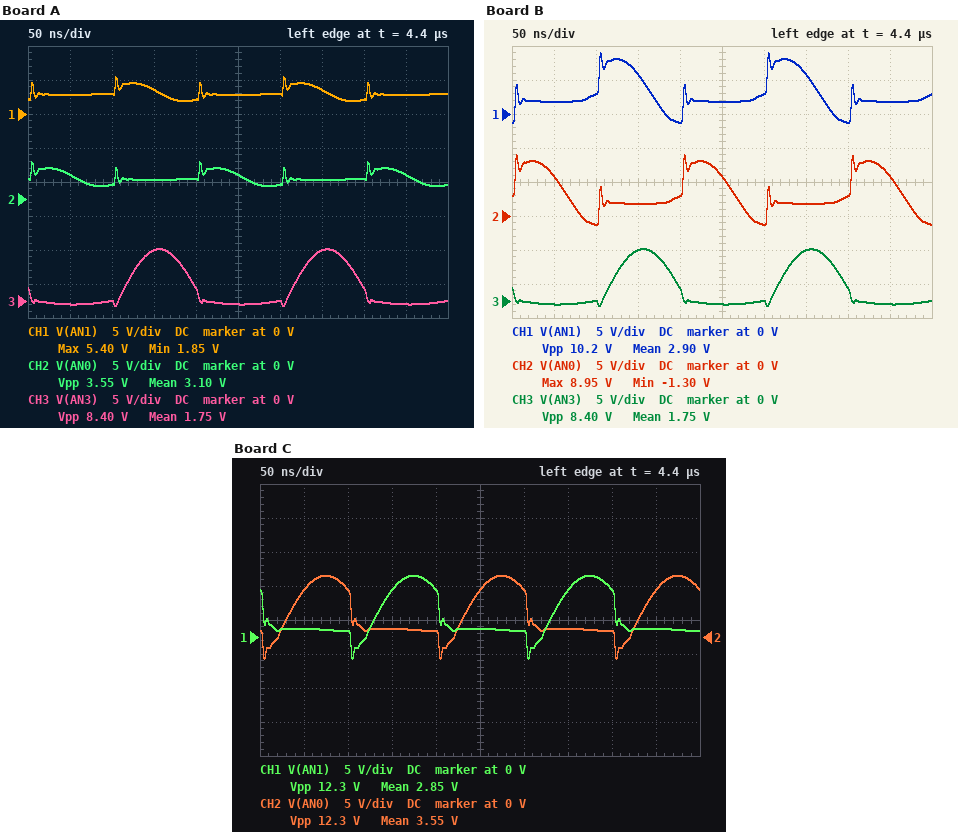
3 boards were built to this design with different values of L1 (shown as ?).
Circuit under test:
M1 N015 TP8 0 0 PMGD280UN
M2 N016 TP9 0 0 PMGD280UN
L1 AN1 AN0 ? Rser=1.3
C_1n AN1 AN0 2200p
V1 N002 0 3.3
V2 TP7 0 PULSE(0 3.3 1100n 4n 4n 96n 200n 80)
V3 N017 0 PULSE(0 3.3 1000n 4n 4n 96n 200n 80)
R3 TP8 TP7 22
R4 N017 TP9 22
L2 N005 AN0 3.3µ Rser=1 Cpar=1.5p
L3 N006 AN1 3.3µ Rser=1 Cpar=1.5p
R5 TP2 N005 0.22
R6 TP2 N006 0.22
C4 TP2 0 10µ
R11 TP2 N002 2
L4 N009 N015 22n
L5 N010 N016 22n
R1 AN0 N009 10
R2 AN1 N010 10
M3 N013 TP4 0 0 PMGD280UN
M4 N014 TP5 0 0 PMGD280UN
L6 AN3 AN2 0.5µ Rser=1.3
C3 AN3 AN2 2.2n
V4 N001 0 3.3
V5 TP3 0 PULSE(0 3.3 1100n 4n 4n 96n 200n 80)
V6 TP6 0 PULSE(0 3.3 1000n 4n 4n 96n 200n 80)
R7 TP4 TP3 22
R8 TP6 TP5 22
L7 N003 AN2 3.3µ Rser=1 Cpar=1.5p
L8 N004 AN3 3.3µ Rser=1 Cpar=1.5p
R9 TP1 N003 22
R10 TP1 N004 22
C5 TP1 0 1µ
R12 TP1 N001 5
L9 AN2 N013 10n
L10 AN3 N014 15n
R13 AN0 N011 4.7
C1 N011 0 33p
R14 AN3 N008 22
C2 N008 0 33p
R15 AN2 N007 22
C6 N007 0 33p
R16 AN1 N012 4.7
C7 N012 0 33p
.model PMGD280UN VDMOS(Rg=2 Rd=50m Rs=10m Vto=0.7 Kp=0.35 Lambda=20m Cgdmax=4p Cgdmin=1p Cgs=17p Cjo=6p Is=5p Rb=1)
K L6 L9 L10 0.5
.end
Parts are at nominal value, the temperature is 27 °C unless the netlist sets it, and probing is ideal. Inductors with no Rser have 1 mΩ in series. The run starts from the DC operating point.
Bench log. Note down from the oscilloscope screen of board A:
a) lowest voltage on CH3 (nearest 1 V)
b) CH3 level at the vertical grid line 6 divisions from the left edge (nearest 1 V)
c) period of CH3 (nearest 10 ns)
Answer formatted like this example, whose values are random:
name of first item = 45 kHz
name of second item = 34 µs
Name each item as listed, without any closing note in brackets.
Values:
lowest voltage on CH3 = -1 V
CH3 level at the vertical grid line 6 divisions from the left edge = 0 V
period of CH3 = 200 ns
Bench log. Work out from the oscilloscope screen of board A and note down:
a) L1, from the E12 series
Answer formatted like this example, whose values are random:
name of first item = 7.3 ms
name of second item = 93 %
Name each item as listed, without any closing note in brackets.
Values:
L1, from the E12 series = 180 nH
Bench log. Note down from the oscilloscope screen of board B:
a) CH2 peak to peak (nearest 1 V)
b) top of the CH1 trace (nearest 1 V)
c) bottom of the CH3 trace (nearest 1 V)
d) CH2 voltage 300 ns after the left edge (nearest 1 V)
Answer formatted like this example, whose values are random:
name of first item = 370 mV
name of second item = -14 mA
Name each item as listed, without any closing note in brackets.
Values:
CH2 peak to peak = 10 V
top of the CH1 trace = 9 V
bottom of the CH3 trace = -1 V
CH2 voltage 300 ns after the left edge = -1 V
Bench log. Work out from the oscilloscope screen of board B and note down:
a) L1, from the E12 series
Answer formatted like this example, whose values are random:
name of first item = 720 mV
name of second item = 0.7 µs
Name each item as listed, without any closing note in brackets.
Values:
L1, from the E12 series = 390 nH
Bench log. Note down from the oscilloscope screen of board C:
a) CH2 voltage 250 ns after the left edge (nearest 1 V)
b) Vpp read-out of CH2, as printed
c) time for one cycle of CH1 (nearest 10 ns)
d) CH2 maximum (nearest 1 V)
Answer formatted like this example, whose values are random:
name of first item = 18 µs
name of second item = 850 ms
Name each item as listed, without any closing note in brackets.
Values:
CH2 voltage 250 ns after the left edge = 7 V
Vpp read-out of CH2, as printed = 12.3 V
time for one cycle of CH1 = 200 ns
CH2 maximum = 9 V
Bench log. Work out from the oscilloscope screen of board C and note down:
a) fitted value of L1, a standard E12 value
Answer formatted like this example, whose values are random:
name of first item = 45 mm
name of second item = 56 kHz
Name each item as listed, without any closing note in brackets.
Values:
fitted value of L1, a standard E12 value = 560 nH
